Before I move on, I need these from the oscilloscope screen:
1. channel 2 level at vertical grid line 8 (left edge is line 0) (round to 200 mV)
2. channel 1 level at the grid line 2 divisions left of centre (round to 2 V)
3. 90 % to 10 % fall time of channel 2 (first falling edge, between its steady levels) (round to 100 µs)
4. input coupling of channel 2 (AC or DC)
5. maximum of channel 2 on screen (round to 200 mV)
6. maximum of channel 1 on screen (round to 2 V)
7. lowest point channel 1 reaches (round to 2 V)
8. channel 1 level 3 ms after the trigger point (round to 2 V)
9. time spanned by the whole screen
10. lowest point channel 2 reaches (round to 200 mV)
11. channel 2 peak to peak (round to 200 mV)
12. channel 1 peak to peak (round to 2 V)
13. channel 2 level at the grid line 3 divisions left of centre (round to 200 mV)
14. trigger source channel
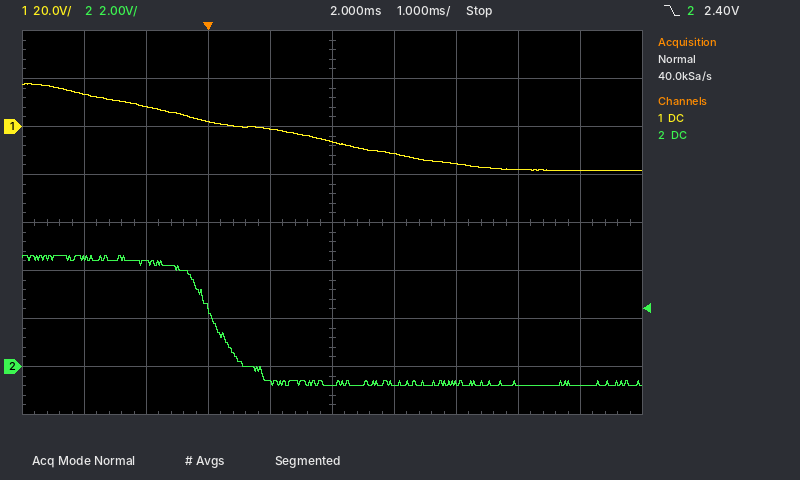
-800 mV
2 V
1.2 ms
DC
4.6 V
18 V
-18 V
-12 V
10 ms
-800 mV
5.4 V
36 V
4.4 V
channel 2
